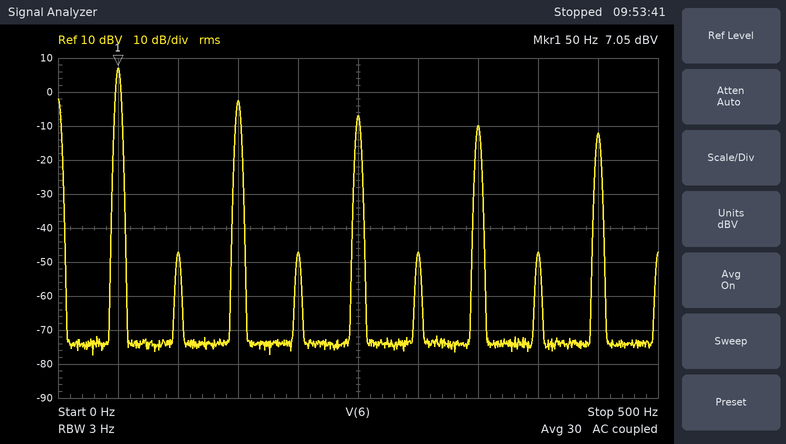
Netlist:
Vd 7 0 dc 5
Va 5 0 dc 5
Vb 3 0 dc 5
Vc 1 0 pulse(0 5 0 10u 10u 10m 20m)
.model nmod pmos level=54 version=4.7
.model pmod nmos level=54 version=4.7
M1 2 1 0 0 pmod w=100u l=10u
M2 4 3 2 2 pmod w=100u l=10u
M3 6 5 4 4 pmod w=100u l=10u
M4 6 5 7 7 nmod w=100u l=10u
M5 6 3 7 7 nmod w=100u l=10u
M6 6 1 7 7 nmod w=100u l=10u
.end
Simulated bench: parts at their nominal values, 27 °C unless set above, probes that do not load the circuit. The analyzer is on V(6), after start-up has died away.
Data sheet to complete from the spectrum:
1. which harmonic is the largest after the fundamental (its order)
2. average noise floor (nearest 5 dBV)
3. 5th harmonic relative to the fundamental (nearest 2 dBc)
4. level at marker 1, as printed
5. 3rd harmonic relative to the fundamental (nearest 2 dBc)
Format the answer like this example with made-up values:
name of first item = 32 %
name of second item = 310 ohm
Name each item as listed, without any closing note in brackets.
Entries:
which harmonic is the largest after the fundamental = 3
average noise floor = -75 dBV
5th harmonic relative to the fundamental = -14 dBc
level at marker 1, as printed = 7.05 dBV
3rd harmonic relative to the fundamental = -10 dBc
